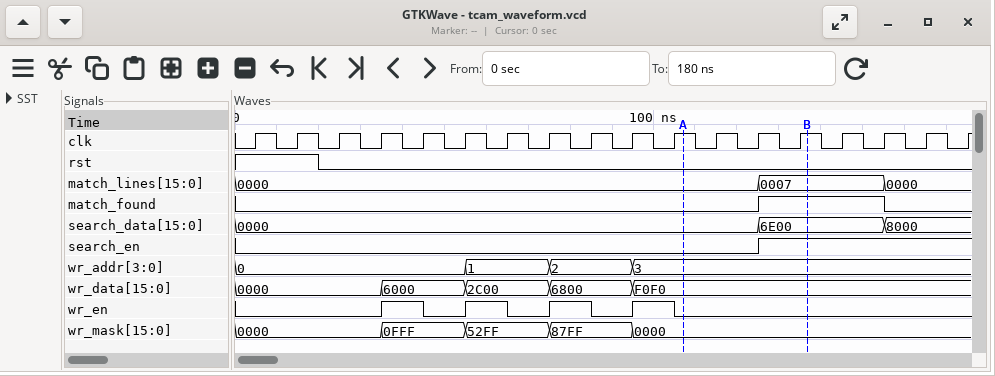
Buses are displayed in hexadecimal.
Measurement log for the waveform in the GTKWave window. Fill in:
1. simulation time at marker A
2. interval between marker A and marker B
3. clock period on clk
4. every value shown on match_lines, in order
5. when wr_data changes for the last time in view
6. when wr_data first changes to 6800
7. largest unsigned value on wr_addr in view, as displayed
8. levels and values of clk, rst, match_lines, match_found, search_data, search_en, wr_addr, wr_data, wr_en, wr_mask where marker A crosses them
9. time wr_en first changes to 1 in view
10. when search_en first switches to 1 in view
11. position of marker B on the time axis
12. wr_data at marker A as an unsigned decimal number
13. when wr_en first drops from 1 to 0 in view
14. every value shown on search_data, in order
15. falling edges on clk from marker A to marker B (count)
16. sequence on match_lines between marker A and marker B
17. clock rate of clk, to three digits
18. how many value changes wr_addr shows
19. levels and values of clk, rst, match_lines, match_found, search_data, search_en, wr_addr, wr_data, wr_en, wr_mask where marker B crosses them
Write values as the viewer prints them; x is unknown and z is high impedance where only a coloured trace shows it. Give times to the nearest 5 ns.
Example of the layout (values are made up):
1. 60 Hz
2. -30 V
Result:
1. 105 ns
2. 30 ns
3. 10 ns
4. 0000, 0007, 0000
5. 95 ns
6. 75 ns
7. 3
8. clk=1, rst=0, match_lines=0000, match_found=0, search_data=0000, search_en=0, wr_addr=3, wr_data=F0F0, wr_en=0, wr_mask=0000
9. 35 ns
10. 125 ns
11. 135 ns
12. 61680
13. 45 ns
14. 0000, 6E00, 8000
15. 3
16. 0000, 0007
17. 100 MHz
18. 3
19. clk=1, rst=0, match_lines=0007, match_found=1, search_data=6E00, search_en=1, wr_addr=3, wr_data=F0F0, wr_en=0, wr_mask=0000
